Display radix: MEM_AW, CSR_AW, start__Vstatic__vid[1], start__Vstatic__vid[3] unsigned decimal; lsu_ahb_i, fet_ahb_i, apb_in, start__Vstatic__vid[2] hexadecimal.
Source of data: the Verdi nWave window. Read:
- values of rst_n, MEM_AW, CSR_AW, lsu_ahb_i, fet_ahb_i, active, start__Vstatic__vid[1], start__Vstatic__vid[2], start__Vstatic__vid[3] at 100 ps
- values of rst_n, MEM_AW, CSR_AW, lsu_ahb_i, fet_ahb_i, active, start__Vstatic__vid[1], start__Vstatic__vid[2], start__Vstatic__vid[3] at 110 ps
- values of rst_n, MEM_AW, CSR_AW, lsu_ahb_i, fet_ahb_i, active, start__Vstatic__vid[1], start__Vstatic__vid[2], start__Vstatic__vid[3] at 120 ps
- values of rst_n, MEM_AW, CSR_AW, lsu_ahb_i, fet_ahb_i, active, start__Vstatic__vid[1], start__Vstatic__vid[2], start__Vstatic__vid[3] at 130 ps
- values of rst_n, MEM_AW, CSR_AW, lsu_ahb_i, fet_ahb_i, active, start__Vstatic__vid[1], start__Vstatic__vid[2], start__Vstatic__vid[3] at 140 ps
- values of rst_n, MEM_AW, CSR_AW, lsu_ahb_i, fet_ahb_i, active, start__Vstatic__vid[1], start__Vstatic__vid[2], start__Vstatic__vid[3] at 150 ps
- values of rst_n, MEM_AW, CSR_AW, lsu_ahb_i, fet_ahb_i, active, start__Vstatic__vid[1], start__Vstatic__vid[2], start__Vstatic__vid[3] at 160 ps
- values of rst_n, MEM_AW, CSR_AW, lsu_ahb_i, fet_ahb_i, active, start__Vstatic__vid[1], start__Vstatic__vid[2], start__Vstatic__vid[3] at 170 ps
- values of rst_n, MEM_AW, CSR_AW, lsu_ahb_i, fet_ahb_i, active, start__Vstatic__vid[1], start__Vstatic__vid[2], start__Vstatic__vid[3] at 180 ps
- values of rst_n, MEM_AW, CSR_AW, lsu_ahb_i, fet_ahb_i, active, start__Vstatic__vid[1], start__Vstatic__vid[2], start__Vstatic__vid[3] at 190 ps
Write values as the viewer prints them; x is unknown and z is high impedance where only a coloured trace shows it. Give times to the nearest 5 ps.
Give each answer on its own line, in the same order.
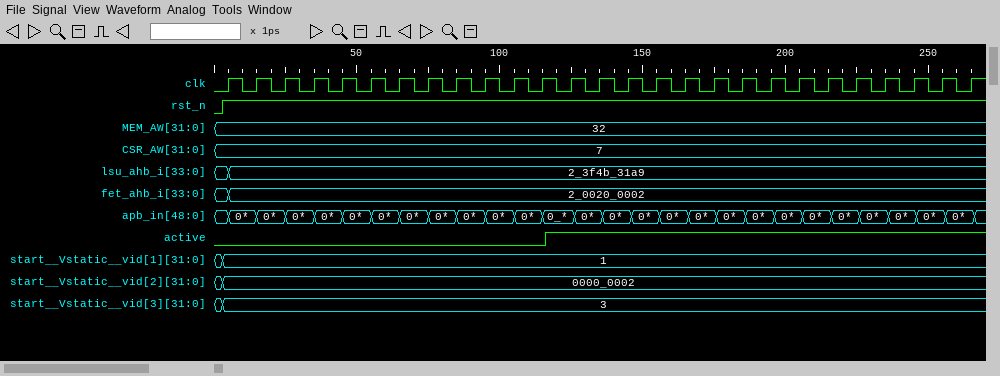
rst_n=1, MEM_AW=32, CSR_AW=7, lsu_ahb_i=2_3f4b_31a9, fet_ahb_i=2_0020_0002, active=0, start__Vstatic__vid[1]=1, start__Vstatic__vid[2]=0000_0002, start__Vstatic__vid[3]=3
rst_n=1, MEM_AW=32, CSR_AW=7, lsu_ahb_i=2_3f4b_31a9, fet_ahb_i=2_0020_0002, active=0, start__Vstatic__vid[1]=1, start__Vstatic__vid[2]=0000_0002, start__Vstatic__vid[3]=3
rst_n=1, MEM_AW=32, CSR_AW=7, lsu_ahb_i=2_3f4b_31a9, fet_ahb_i=2_0020_0002, active=1, start__Vstatic__vid[1]=1, start__Vstatic__vid[2]=0000_0002, start__Vstatic__vid[3]=3
rst_n=1, MEM_AW=32, CSR_AW=7, lsu_ahb_i=2_3f4b_31a9, fet_ahb_i=2_0020_0002, active=1, start__Vstatic__vid[1]=1, start__Vstatic__vid[2]=0000_0002, start__Vstatic__vid[3]=3
rst_n=1, MEM_AW=32, CSR_AW=7, lsu_ahb_i=2_3f4b_31a9, fet_ahb_i=2_0020_0002, active=1, start__Vstatic__vid[1]=1, start__Vstatic__vid[2]=0000_0002, start__Vstatic__vid[3]=3
rst_n=1, MEM_AW=32, CSR_AW=7, lsu_ahb_i=2_3f4b_31a9, fet_ahb_i=2_0020_0002, active=1, start__Vstatic__vid[1]=1, start__Vstatic__vid[2]=0000_0002, start__Vstatic__vid[3]=3
rst_n=1, MEM_AW=32, CSR_AW=7, lsu_ahb_i=2_3f4b_31a9, fet_ahb_i=2_0020_0002, active=1, start__Vstatic__vid[1]=1, start__Vstatic__vid[2]=0000_0002, start__Vstatic__vid[3]=3
rst_n=1, MEM_AW=32, CSR_AW=7, lsu_ahb_i=2_3f4b_31a9, fet_ahb_i=2_0020_0002, active=1, start__Vstatic__vid[1]=1, start__Vstatic__vid[2]=0000_0002, start__Vstatic__vid[3]=3
rst_n=1, MEM_AW=32, CSR_AW=7, lsu_ahb_i=2_3f4b_31a9, fet_ahb_i=2_0020_0002, active=1, start__Vstatic__vid[1]=1, start__Vstatic__vid[2]=0000_0002, start__Vstatic__vid[3]=3
rst_n=1, MEM_AW=32, CSR_AW=7, lsu_ahb_i=2_3f4b_31a9, fet_ahb_i=2_0020_0002, active=1, start__Vstatic__vid[1]=1, start__Vstatic__vid[2]=0000_0002, start__Vstatic__vid[3]=3
